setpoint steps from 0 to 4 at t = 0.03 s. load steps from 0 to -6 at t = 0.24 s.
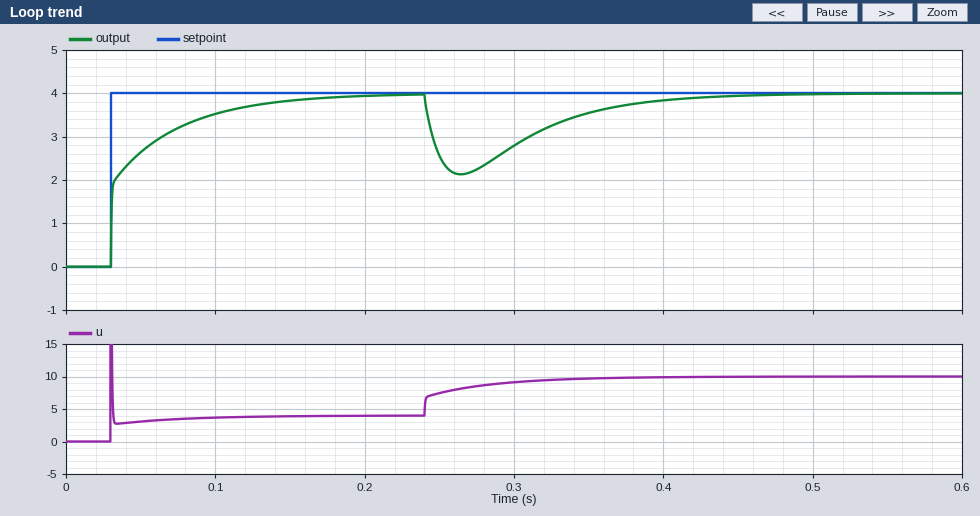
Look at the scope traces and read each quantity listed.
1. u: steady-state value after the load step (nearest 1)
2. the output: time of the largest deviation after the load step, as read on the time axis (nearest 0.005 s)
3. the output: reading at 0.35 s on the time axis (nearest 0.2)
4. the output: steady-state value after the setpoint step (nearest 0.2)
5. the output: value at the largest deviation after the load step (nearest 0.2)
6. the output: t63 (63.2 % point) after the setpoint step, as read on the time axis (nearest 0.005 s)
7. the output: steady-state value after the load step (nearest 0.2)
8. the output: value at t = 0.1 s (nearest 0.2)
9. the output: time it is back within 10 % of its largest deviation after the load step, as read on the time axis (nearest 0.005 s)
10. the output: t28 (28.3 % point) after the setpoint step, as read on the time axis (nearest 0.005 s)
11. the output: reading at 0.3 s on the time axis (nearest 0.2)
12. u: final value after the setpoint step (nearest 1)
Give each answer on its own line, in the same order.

10
0.265 s
3.6
4.0
2.2
0.045 s
4.0
3.6
0.395 s
0.030 s
2.8
4
